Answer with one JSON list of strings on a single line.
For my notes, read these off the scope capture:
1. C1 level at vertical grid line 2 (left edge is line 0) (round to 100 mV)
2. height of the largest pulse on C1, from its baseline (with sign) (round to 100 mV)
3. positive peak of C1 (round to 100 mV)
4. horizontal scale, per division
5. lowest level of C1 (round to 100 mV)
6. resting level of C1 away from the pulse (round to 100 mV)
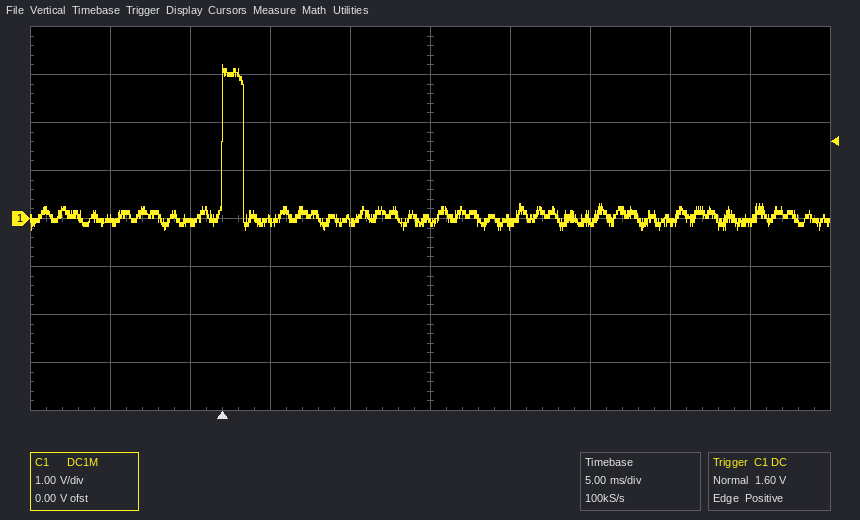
["-100 mV", "+3.2 V", "3.2 V", "5 ms", "-200 mV", "0.0 V"]
